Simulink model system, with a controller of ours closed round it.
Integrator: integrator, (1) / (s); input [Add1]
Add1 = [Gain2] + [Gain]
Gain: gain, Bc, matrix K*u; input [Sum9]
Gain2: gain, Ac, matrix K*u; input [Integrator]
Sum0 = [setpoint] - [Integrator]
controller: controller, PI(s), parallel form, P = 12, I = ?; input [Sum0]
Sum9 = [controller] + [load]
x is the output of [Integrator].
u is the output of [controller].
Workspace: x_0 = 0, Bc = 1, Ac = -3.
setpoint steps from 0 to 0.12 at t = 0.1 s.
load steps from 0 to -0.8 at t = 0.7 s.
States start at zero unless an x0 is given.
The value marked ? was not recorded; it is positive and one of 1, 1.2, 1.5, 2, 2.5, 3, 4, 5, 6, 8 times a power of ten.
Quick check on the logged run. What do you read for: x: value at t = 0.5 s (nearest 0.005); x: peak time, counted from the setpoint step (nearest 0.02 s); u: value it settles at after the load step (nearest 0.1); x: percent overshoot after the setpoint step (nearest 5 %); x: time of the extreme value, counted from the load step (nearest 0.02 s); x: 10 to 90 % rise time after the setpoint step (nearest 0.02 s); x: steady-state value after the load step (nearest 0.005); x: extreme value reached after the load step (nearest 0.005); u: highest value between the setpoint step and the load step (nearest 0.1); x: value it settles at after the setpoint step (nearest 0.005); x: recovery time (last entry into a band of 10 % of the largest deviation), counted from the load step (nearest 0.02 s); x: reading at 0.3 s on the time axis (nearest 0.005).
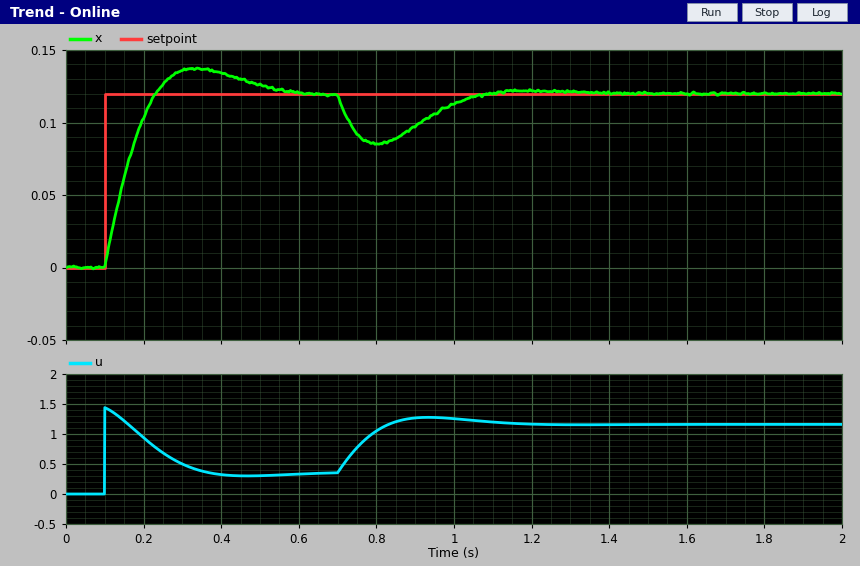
0.125
0.24 s
1.2
15 %
0.10 s
0.10 s
0.120
0.085
1.4
0.120
0.34 s
0.135
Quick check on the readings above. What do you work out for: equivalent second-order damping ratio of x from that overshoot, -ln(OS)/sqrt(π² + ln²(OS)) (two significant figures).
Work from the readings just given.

0.52
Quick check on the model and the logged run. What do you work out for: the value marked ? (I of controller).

120
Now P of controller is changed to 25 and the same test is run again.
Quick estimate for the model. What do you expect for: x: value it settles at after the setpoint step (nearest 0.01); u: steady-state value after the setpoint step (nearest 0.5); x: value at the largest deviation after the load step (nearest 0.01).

0.12
0.5
0.10
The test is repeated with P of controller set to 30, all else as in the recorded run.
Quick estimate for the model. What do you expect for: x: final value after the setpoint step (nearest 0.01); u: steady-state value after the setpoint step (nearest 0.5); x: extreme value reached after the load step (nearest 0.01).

0.12
0.5
0.10
